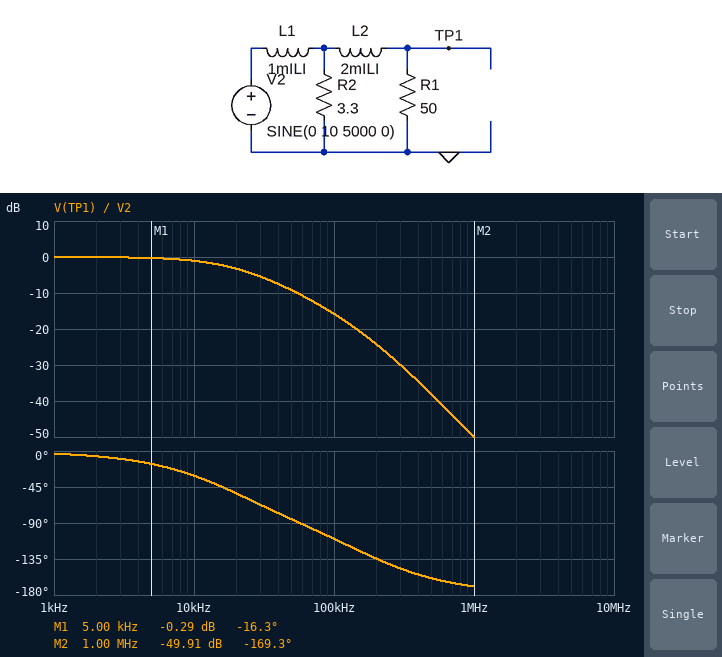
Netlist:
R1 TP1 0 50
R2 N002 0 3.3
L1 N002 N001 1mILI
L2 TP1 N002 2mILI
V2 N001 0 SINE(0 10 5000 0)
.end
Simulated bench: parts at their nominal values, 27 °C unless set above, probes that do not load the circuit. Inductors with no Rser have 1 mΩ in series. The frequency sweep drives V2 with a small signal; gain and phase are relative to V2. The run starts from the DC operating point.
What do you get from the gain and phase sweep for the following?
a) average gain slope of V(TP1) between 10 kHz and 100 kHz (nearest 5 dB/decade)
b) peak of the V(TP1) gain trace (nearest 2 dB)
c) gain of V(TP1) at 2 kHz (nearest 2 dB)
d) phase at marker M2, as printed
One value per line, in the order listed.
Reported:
-15 dB/decade
0 dB
0 dB
-169.3 deg
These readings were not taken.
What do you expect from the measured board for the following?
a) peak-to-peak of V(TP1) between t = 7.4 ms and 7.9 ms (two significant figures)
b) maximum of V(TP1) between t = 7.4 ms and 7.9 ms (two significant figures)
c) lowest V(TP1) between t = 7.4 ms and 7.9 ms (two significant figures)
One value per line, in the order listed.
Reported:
19 V
9.7 V
-9.7 V
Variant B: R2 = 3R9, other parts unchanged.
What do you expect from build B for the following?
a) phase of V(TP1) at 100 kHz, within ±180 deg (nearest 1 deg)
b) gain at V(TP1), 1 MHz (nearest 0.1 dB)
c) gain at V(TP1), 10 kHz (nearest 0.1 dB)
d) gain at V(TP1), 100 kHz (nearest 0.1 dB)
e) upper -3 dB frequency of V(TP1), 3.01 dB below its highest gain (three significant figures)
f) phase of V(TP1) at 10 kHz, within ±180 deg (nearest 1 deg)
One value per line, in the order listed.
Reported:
-108 deg
-48.5 dB
-0.8 dB
-14.5 dB
22.0 kHz
-27 deg
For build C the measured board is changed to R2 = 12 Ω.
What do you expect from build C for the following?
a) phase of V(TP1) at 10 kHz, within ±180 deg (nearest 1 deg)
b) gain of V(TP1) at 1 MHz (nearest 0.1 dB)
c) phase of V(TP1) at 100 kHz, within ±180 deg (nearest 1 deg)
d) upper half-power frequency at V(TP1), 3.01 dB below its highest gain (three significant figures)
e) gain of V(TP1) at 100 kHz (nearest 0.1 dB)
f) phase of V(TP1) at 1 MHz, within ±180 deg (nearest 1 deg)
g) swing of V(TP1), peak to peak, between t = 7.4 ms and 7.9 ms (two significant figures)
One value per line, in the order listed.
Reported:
-13 deg
-38.8 dB
-86 deg
51.8 kHz
-7.2 dB
-165 deg
20 V
